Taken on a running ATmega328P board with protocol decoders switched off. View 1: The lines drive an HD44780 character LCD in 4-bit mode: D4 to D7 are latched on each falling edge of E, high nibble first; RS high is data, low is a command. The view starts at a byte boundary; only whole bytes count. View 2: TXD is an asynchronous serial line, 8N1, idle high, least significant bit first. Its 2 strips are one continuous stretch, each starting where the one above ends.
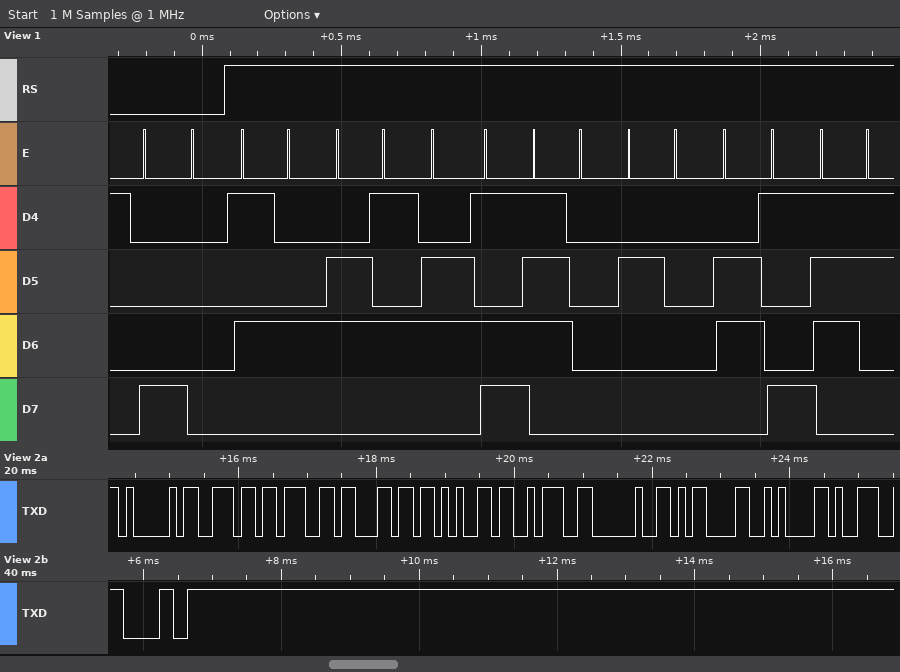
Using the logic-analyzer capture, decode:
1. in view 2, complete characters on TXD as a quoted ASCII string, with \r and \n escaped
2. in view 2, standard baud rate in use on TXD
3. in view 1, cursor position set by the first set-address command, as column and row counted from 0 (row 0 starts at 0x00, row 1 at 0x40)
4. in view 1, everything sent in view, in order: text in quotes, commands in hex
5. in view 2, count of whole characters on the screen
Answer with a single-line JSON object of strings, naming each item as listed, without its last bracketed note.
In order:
{"in view 2, complete characters on TXD as a quoted ASCII string, with \\r and \\n escaped": "\"Angle: \\r\\n90\"", "in view 2, standard baud rate in use on TXD": "9600 baud", "in view 1, cursor position set by the first set-address command, as column and row counted from 0": "column 0, row 0", "in view 1, everything sent in view, in order: text in quotes, commands in hex": "0x80 \"Temp is\"", "in view 2, count of whole characters on the screen": "11"}
